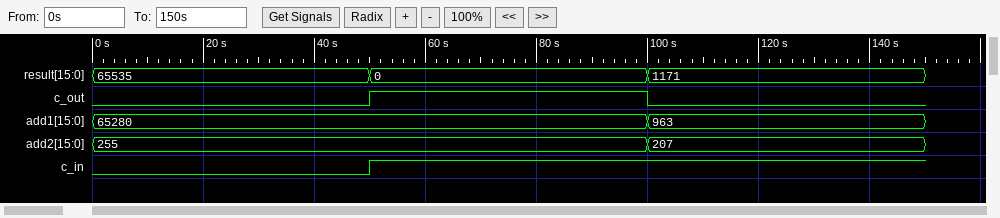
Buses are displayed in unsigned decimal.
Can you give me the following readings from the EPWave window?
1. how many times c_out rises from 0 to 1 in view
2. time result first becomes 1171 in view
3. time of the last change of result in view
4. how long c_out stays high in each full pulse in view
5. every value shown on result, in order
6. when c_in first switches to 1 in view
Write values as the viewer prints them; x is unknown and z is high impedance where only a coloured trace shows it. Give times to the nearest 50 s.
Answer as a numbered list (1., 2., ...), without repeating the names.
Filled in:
1. 1
2. 100 s
3. 100 s
4. 50 s
5. 65535, 0, 1171
6. 50 s
